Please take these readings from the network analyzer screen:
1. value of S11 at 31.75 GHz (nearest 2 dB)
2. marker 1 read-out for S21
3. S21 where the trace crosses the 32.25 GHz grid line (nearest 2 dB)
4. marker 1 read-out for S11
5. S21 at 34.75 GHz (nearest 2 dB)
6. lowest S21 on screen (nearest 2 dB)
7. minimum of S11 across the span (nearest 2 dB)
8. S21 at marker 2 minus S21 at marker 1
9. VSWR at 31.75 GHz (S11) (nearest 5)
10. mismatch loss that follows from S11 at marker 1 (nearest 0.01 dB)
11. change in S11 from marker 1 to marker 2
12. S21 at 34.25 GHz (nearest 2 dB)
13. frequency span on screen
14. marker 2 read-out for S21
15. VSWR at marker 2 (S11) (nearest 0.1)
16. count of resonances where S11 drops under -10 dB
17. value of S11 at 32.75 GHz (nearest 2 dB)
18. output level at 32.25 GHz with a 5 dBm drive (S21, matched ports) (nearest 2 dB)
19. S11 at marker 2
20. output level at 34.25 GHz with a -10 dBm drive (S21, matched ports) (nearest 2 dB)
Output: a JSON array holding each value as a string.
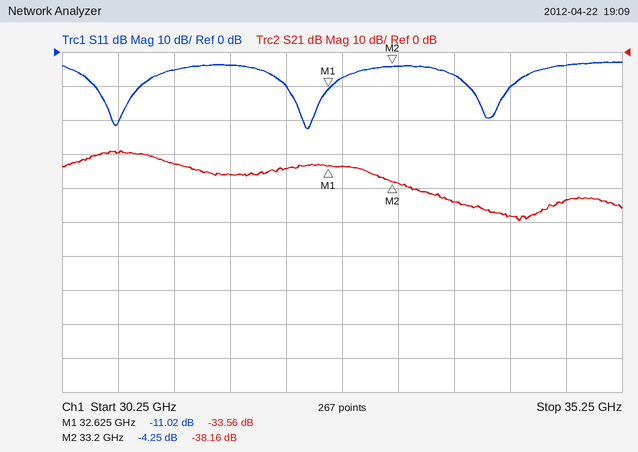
["-4 dB", "-33.56 dB", "-34 dB", "-11.02 dB", "-44 dB", "-50 dB", "-22 dB", "-4.60 dB", "5", "0.36 dB", "6.77 dB", "-48 dB", "5 GHz", "-38.16 dB", "4.2", "3", "-8 dB", "-30 dBm", "-4.25 dB", "-58 dBm"]
